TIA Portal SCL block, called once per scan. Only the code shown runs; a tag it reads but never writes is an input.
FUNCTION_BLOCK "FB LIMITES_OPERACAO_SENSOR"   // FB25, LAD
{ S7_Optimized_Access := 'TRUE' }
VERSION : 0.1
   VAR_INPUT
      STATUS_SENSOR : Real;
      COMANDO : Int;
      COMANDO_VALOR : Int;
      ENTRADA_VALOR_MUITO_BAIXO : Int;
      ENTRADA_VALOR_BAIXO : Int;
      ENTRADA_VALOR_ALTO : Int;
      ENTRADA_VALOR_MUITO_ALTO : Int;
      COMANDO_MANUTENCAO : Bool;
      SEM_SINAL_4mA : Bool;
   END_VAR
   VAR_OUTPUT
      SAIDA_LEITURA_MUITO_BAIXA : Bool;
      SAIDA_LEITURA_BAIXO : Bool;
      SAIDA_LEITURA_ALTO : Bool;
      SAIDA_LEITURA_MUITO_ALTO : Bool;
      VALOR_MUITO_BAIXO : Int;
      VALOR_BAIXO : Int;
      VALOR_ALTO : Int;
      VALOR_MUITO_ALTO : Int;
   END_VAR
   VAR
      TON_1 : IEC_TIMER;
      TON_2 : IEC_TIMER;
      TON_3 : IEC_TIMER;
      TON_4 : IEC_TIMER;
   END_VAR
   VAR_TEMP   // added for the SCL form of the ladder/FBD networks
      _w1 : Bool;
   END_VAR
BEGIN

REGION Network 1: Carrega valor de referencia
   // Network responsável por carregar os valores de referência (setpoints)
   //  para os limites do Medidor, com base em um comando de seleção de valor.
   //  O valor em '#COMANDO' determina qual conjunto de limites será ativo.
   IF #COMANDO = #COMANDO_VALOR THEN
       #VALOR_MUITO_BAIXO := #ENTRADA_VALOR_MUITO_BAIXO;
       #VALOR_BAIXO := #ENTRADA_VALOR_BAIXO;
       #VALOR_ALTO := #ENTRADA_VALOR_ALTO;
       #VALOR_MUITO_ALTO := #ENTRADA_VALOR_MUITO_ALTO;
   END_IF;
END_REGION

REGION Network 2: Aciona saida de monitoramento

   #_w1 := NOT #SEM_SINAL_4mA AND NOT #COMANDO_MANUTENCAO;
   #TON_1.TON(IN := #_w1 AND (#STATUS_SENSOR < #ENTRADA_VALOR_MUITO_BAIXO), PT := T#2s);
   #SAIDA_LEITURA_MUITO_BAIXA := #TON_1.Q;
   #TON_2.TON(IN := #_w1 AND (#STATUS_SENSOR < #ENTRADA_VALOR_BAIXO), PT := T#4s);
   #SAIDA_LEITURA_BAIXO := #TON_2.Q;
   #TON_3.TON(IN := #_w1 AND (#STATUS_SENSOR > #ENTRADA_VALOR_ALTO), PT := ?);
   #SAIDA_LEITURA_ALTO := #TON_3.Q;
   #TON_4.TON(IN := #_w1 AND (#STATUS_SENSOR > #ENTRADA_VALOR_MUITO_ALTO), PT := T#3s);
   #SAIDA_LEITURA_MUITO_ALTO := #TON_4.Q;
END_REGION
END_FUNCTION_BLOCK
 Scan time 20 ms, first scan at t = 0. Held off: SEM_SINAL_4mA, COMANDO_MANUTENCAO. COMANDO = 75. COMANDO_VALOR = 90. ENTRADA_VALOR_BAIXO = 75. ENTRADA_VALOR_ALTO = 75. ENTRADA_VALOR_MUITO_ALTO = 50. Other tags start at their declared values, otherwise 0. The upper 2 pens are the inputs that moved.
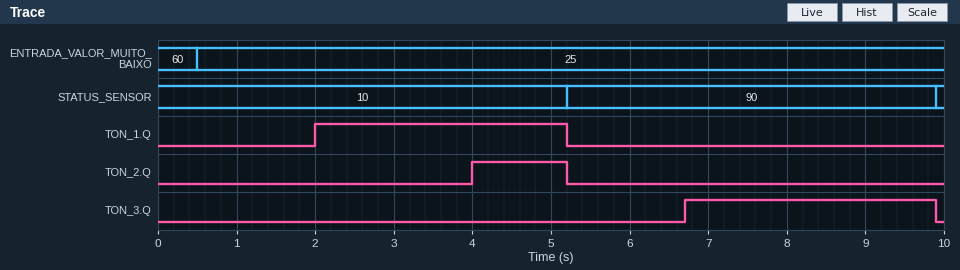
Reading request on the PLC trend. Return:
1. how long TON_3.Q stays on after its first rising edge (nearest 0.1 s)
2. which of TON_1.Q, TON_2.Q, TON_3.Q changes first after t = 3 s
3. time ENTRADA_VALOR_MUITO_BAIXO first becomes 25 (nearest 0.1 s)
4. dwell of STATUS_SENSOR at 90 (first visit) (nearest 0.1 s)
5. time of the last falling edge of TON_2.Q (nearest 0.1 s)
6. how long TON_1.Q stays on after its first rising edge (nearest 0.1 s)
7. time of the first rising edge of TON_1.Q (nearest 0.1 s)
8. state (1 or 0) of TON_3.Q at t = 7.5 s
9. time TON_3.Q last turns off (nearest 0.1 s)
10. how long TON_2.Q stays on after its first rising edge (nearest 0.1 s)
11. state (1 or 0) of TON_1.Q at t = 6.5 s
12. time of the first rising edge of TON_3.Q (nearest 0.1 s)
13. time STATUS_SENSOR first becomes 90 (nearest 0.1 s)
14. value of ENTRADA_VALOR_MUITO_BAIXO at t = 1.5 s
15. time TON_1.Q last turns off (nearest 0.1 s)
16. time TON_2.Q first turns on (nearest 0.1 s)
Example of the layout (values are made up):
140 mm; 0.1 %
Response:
3.2 s; TON_2.Q; 0.5 s; 4.7 s; 5.2 s; 3.2 s; 2.0 s; 1; 9.9 s; 1.2 s; 0; 6.7 s; 5.2 s; 25; 5.2 s; 4.0 s
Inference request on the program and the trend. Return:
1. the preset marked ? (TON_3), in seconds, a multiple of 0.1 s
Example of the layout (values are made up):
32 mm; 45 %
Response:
1.5 s
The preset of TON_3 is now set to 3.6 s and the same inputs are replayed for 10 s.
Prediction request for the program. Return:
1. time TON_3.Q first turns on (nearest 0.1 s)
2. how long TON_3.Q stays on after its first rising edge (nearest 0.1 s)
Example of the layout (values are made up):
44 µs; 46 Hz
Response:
8.8 s; 1.1 s
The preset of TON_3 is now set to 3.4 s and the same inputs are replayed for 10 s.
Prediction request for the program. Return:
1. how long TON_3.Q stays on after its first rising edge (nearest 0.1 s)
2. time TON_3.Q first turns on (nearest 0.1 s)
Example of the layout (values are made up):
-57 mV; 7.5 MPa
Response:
1.3 s; 8.6 s
